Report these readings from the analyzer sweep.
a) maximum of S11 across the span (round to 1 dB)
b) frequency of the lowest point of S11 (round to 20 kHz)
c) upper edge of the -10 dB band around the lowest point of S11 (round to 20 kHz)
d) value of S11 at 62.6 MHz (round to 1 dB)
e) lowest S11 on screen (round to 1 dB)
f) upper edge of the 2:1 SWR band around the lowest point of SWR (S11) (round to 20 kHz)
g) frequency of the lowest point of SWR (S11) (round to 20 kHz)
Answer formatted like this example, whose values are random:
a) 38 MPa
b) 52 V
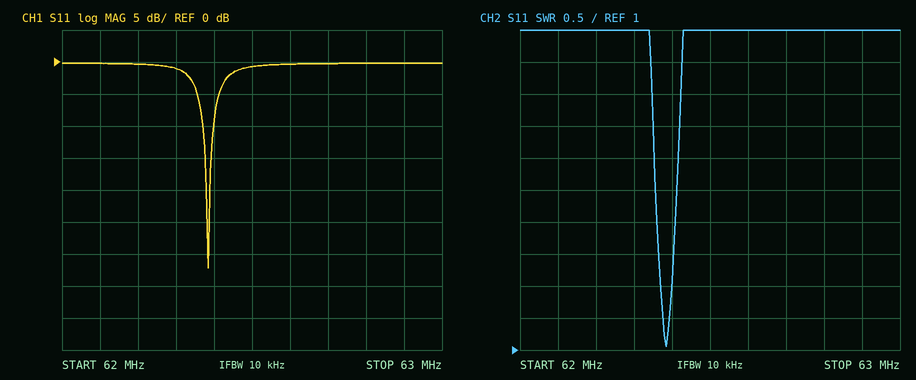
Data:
a) 0 dB
b) 62.38 MHz
c) 62.40 MHz
d) 0 dB
e) -32 dB
f) 62.40 MHz
g) 62.38 MHz
